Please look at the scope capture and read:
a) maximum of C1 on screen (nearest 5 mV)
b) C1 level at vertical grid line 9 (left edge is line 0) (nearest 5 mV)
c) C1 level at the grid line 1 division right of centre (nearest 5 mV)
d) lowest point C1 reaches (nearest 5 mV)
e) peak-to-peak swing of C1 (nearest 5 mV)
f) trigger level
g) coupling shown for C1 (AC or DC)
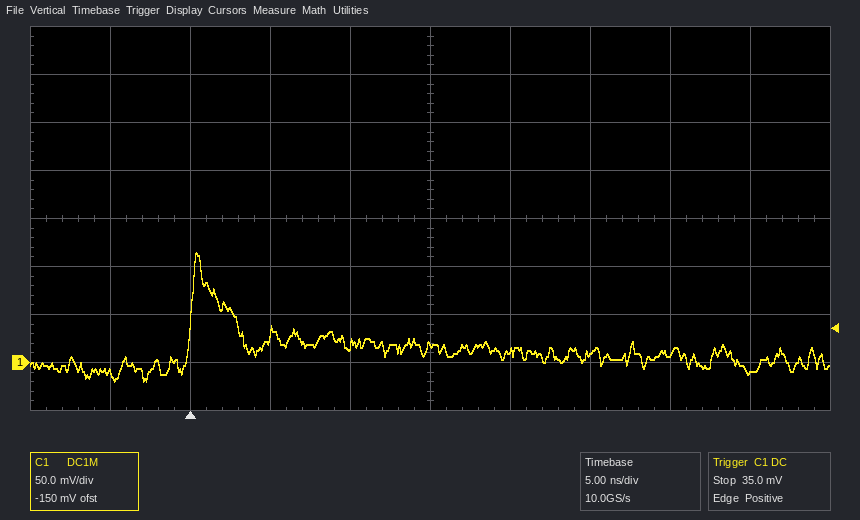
115 mV
-10 mV
10 mV
-20 mV
135 mV
35.0 mV
DC
